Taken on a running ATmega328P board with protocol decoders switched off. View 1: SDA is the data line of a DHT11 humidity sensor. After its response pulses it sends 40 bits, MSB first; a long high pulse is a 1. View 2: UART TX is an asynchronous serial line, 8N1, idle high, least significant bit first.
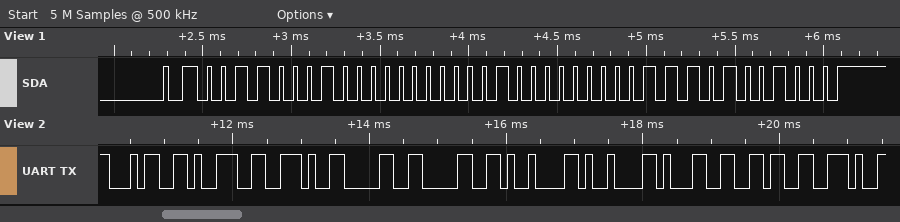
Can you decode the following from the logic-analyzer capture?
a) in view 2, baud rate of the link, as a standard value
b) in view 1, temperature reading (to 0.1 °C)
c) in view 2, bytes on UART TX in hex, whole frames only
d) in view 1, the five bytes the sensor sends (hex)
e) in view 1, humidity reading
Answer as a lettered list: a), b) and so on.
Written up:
a) 9600 baud
b) 16.7 °C
c) 34 39 2E 30 30 09 09 31 36 2E
d) 31 00 10 07 48
e) 49 %
